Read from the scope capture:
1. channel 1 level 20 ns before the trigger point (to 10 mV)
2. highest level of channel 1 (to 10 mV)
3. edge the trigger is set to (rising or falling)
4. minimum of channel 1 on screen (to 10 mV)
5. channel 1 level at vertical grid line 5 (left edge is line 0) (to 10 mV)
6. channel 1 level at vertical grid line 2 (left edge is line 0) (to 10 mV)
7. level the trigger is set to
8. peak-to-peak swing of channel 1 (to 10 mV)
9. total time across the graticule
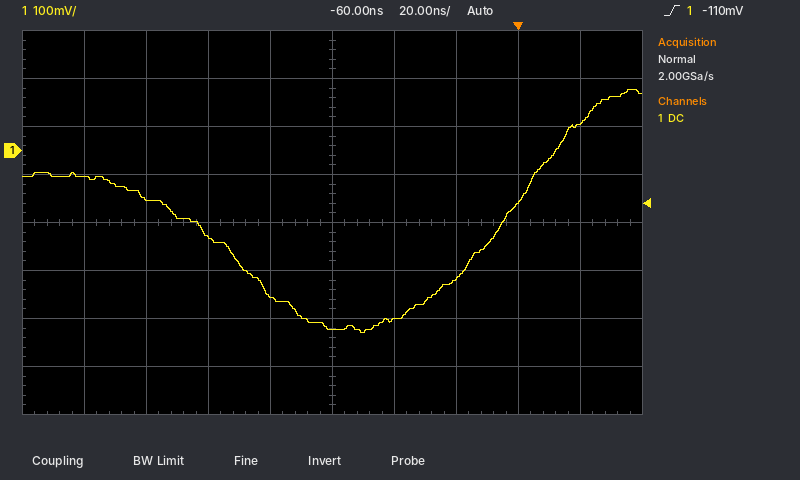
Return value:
-270 mV
130 mV
rising
-380 mV
-370 mV
-100 mV
-110 mV
510 mV
200 ns
